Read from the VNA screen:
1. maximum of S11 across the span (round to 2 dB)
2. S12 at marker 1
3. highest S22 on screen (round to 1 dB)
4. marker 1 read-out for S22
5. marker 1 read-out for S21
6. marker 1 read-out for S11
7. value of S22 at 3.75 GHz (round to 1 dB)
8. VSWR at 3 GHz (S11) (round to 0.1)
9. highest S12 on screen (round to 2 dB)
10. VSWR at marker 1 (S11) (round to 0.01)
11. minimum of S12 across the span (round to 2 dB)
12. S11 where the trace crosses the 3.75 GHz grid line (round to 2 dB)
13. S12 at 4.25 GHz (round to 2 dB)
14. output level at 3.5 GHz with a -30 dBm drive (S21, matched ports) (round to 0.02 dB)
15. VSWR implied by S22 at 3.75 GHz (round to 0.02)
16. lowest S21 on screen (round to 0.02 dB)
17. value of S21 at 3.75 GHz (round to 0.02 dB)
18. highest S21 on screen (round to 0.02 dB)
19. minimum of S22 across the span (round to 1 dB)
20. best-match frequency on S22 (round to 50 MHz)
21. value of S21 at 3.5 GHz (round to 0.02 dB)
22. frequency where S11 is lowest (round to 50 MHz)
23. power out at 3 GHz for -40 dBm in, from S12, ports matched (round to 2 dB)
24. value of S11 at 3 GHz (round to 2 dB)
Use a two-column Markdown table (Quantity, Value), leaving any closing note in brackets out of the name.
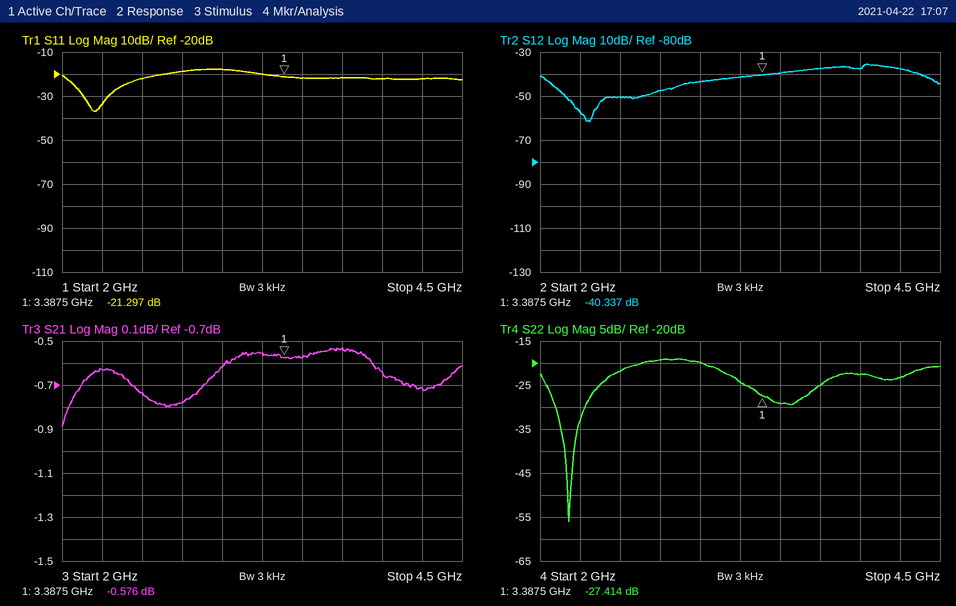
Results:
| Quantity | Value |
|---|---|
| maximum of S11 across the span | -18 dB |
| S12 at marker 1 | -40.337 dB |
| highest S22 on screen | -19 dB |
| marker 1 read-out for S22 | -27.414 dB |
| marker 1 read-out for S21 | -0.576 dB |
| marker 1 read-out for S11 | -21.297 dB |
| value of S22 at 3.75 GHz | -25 dB |
| VSWR at 3 GHz (S11) | 1.3 |
| highest S12 on screen | -36 dB |
| VSWR at marker 1 (S11) | 1.19 |
| minimum of S12 across the span | -62 dB |
| S11 where the trace crosses the 3.75 GHz grid line | -22 dB |
| S12 at 4.25 GHz | -38 dB |
| output level at 3.5 GHz with a -30 dBm drive (S21, matched ports) | -30.58 dBm |
| VSWR implied by S22 at 3.75 GHz | 1.12 |
| lowest S21 on screen | -0.88 dB |
| value of S21 at 3.75 GHz | -0.54 dB |
| highest S21 on screen | -0.54 dB |
| minimum of S22 across the span | -56 dB |
| best-match frequency on S22 | 2.20 GHz |
| value of S21 at 3.5 GHz | -0.58 dB |
| frequency where S11 is lowest | 2.20 GHz |
| power out at 3 GHz for -40 dBm in, from S12, ports matched | -84 dBm |
| value of S11 at 3 GHz | -18 dB |
